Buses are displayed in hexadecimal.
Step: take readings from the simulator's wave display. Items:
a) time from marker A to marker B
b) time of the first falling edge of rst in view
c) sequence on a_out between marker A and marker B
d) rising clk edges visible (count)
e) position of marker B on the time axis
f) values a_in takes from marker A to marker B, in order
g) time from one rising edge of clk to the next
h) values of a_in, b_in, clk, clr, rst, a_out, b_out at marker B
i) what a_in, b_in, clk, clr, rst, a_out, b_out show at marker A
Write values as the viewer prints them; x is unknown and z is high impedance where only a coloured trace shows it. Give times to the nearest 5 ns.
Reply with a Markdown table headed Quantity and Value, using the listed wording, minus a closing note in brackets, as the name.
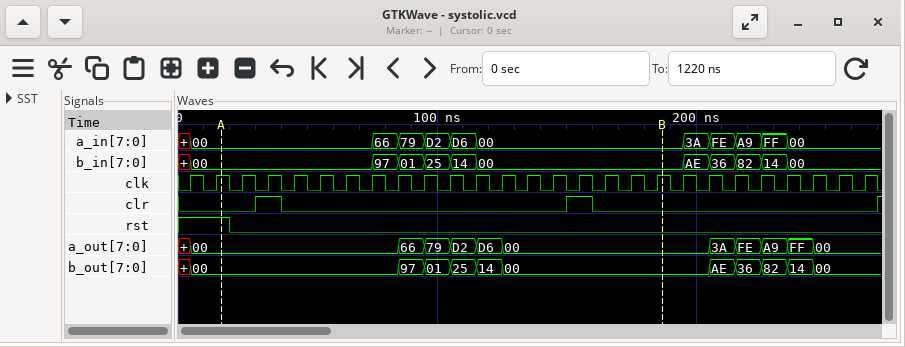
| Quantity | Value |
|---|---|
| time from marker A to marker B | 170 ns |
| time of the first falling edge of rst in view | 20 ns |
| sequence on a_out between marker A and marker B | 00, 66, 79, D2, D6, 00 |
| rising clk edges visible | 27 |
| position of marker B on the time axis | 185 ns |
| values a_in takes from marker A to marker B, in order | 00, 66, 79, D2, D6, 00 |
| time from one rising edge of clk to the next | 10 ns |
| values of a_in, b_in, clk, clr, rst, a_out, b_out at marker B | a_in=00, b_in=00, clk=1, clr=0, rst=0, a_out=00, b_out=00 |
| what a_in, b_in, clk, clr, rst, a_out, b_out show at marker A | a_in=00, b_in=00, clk=1, clr=0, rst=1, a_out=00, b_out=00 |
